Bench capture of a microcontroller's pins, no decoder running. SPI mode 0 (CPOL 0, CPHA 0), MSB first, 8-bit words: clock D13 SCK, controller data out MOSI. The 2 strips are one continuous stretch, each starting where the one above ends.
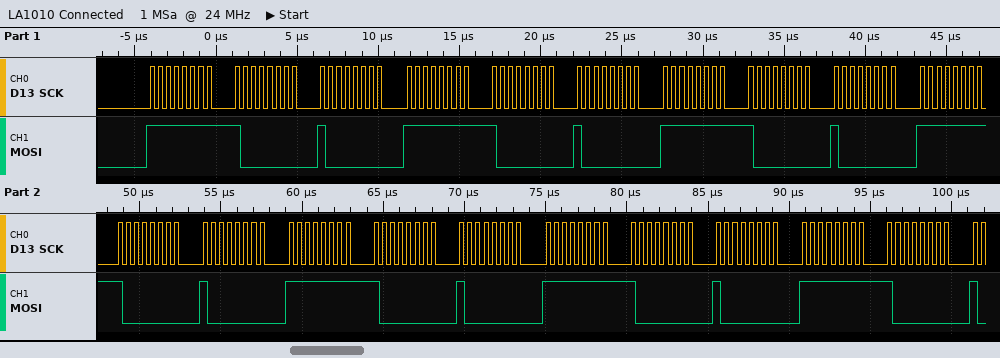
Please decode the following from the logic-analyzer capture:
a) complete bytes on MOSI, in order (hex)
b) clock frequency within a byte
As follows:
FF 80 80 FF 80 80 FF 80 80 FF 80 80 FF 80 80 FF 80 80 FF 80
2 MHz
